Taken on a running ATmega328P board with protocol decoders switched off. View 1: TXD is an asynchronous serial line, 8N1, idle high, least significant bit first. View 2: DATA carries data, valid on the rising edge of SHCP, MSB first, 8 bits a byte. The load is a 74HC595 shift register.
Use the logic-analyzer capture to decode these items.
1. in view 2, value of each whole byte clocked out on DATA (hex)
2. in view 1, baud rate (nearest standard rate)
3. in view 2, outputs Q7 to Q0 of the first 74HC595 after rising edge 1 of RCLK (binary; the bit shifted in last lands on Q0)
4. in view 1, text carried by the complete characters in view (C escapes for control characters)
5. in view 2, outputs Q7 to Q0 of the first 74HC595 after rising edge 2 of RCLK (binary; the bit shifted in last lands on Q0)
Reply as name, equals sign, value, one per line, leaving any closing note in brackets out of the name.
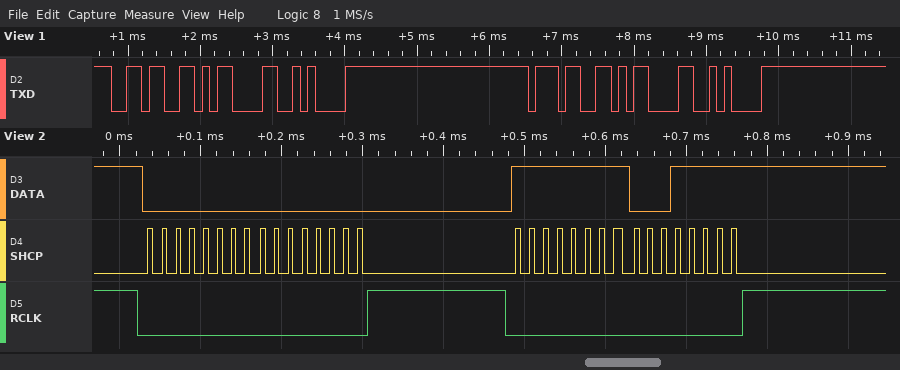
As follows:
in view 2, value of each whole byte clocked out on DATA = 00 00 FF 1F
in view 1, baud rate = 9600 baud
in view 2, outputs Q7 to Q0 of the first 74HC595 after rising edge 1 of RCLK = 00000000
in view 1, text carried by the complete characters in view = "6\r\n7\r\n"
in view 2, outputs Q7 to Q0 of the first 74HC595 after rising edge 2 of RCLK = 00011111
